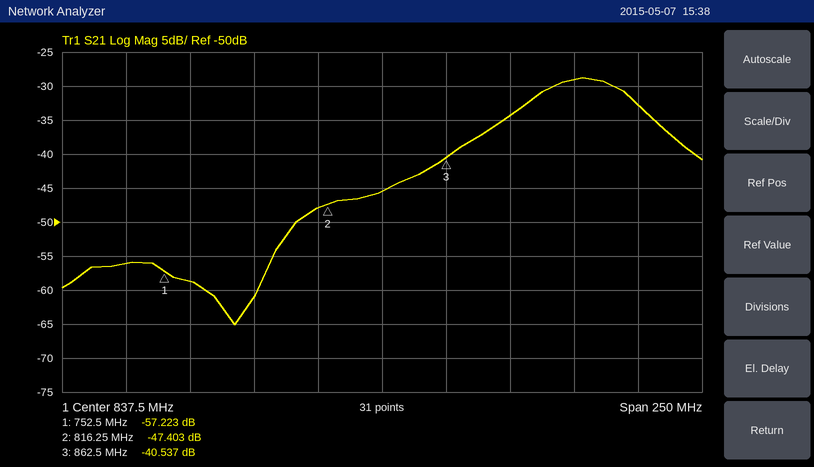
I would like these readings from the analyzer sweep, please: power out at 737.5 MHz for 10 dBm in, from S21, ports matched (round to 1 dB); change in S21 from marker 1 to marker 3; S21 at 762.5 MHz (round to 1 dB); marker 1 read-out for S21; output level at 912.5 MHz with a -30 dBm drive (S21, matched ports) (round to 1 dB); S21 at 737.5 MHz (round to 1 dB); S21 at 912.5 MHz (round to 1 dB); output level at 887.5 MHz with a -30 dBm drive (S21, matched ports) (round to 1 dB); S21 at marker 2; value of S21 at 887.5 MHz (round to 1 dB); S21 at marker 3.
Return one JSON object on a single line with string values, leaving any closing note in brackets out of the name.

{"power out at 737.5 MHz for 10 dBm in, from S21, ports matched": "-46 dBm", "change in S21 from marker 1 to marker 3": "16.686 dB", "S21 at 762.5 MHz": "-59 dB", "marker 1 read-out for S21": "-57.223 dB", "output level at 912.5 MHz with a -30 dBm drive (S21, matched ports)": "-59 dBm", "S21 at 737.5 MHz": "-56 dB", "S21 at 912.5 MHz": "-29 dB", "output level at 887.5 MHz with a -30 dBm drive (S21, matched ports)": "-64 dBm", "S21 at marker 2": "-47.403 dB", "value of S21 at 887.5 MHz": "-34 dB", "S21 at marker 3": "-40.537 dB"}
